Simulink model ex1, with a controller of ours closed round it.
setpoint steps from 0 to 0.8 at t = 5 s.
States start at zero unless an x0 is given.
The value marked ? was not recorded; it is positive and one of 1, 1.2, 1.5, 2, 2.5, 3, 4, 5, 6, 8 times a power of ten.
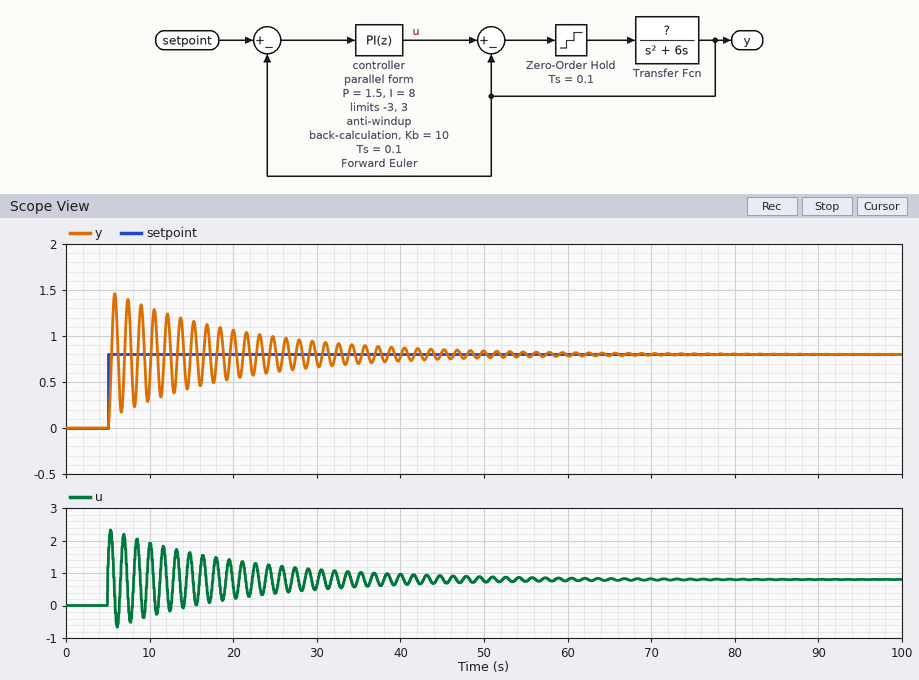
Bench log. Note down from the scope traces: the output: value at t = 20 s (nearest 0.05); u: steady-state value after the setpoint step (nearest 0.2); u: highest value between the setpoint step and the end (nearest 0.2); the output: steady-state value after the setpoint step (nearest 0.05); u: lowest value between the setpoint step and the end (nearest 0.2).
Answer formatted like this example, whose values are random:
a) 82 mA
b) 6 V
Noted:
a) 1.05
b) 0.8
c) 2.4
d) 0.80
e) -0.6
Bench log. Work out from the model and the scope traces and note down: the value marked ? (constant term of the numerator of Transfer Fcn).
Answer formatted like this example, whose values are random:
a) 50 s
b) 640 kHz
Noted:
a) 10
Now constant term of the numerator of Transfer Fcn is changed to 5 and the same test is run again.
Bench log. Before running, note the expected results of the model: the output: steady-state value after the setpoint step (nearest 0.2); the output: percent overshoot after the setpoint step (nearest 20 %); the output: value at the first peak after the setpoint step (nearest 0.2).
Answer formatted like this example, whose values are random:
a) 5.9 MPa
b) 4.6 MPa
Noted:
a) 0.8
b) 80 %
c) 1.4
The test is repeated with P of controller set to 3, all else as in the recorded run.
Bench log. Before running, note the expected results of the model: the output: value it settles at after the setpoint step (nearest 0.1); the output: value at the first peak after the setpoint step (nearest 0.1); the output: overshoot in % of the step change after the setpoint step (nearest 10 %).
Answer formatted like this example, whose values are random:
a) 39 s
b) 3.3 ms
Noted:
a) 0.8
b) 1.3
c) 60 %
